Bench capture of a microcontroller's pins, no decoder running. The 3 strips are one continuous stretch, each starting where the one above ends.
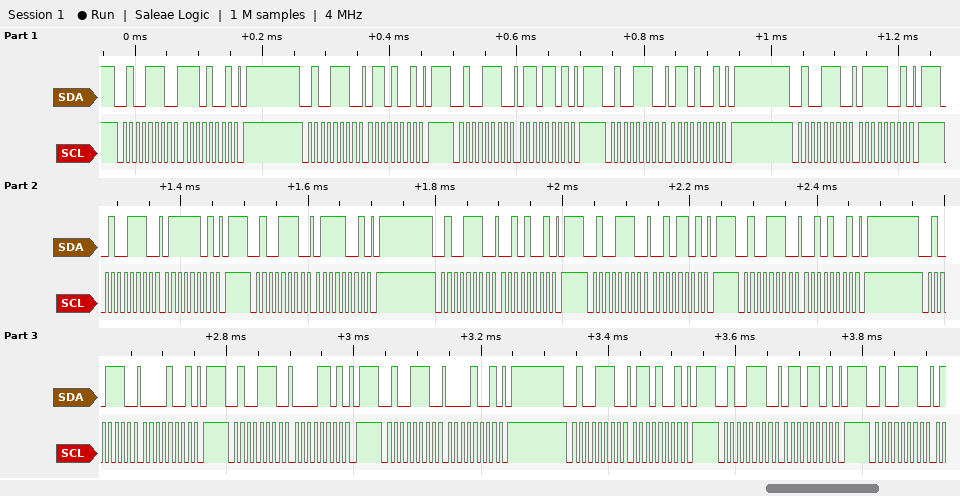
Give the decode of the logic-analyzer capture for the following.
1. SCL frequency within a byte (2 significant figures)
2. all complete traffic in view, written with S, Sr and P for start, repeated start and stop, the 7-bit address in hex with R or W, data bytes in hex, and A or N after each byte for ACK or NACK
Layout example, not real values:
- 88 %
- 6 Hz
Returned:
- 100 kHz
- S 27W A E9 A P S 27W A 69 A P S 27W A 6D A P S 27W A 69 A P S 27W A 79 A P S 27W A 7D A P S 27W A 79 A P S 27W A 29 A P S 27W A 2D A P S 27W A 29 A P S 27W A 09 A P S 27W A 0D A P S 27W A 09 A P S 27W A 69 A P S 27W A 6D A P S 27W A
